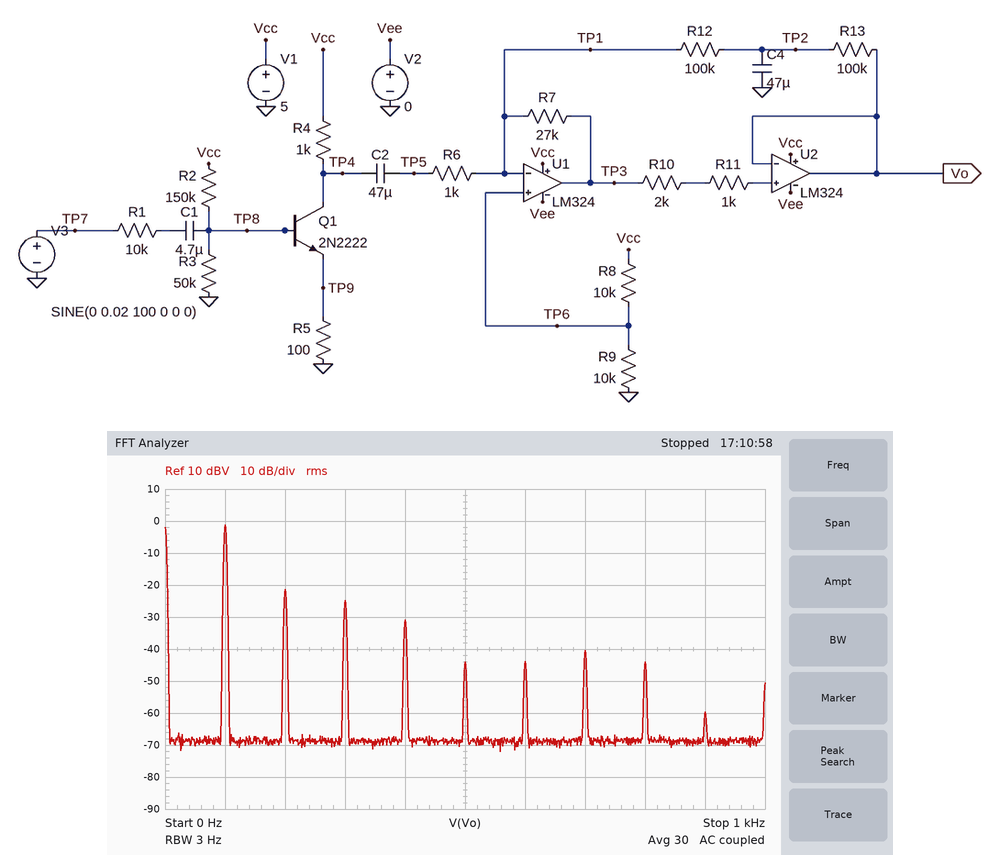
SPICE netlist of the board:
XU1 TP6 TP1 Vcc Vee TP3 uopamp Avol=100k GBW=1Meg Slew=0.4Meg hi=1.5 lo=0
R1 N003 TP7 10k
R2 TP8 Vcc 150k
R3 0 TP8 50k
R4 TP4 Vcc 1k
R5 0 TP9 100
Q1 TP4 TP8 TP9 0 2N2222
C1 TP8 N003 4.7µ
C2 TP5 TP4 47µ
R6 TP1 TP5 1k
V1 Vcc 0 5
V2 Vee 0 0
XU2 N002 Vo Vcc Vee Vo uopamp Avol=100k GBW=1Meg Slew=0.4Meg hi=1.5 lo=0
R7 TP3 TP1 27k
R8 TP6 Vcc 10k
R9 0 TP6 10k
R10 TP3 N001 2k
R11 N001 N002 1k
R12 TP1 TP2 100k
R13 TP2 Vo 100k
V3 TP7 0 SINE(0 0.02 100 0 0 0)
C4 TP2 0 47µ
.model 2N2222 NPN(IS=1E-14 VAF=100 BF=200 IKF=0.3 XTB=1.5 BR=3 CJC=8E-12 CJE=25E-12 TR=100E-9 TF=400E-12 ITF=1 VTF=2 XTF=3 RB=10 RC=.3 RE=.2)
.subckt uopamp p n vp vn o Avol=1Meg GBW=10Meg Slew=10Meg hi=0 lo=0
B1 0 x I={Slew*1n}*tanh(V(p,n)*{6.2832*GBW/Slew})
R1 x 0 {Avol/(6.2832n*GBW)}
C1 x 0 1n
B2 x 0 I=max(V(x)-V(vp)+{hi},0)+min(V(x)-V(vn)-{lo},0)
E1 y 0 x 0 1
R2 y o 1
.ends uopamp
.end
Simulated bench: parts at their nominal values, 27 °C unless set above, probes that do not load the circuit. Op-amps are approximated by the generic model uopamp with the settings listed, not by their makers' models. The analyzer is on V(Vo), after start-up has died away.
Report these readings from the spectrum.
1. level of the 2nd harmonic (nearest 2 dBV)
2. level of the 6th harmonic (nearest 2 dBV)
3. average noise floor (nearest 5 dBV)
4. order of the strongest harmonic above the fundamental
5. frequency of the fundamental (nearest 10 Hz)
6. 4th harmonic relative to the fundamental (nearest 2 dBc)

-22 dBV
-44 dBV
-70 dBV
2
100 Hz
-30 dBc
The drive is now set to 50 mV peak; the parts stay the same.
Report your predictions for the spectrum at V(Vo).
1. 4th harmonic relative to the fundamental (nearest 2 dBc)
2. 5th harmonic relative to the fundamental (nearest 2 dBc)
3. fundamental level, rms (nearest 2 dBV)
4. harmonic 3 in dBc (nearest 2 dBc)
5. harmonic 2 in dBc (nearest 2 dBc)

-22 dBc
-52 dBc
2 dBV
-48 dBc
-8 dBc
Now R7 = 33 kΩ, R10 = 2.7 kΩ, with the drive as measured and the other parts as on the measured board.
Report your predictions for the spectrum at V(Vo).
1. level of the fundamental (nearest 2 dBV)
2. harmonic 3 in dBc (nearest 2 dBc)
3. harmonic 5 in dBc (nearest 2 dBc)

0 dBV
-22 dBc
-34 dBc
